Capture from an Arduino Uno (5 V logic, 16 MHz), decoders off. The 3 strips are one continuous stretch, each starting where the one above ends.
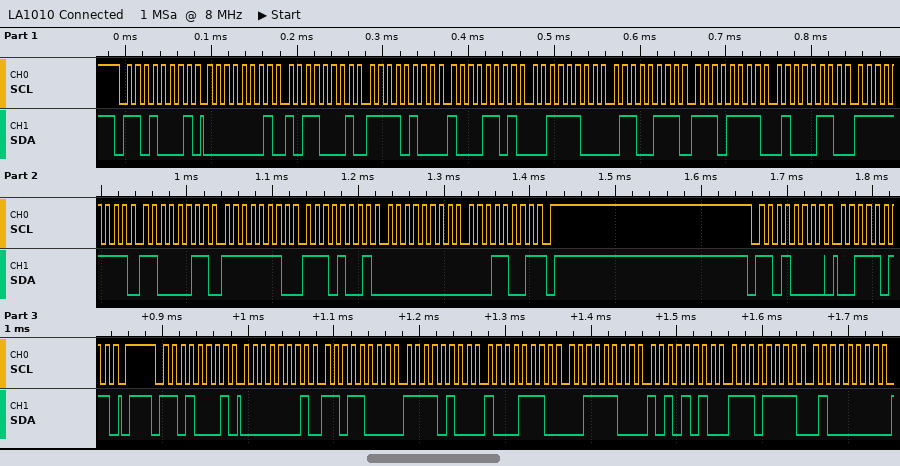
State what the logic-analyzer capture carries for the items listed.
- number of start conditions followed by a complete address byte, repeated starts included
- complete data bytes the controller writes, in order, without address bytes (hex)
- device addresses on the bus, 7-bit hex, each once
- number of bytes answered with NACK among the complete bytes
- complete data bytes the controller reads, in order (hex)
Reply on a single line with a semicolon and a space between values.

3; 3B; 0x68; 1; 01 B1 F4 8D 3C 67 EF 46 FF C3 FE E9 00 19 01 D8 F4 8E 3C AA EF 40
